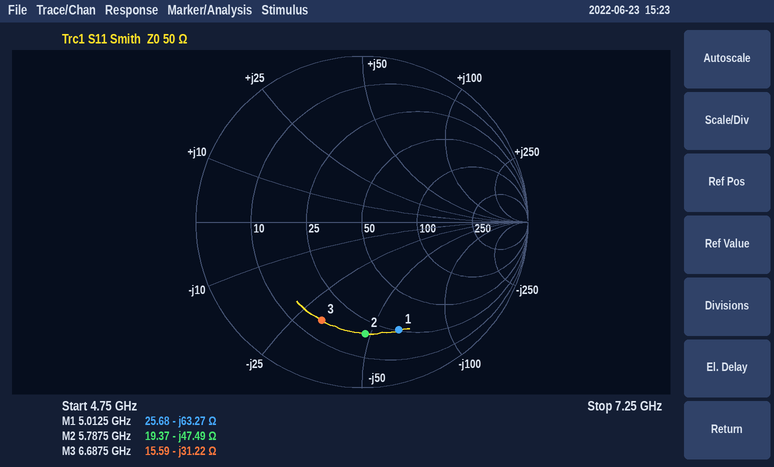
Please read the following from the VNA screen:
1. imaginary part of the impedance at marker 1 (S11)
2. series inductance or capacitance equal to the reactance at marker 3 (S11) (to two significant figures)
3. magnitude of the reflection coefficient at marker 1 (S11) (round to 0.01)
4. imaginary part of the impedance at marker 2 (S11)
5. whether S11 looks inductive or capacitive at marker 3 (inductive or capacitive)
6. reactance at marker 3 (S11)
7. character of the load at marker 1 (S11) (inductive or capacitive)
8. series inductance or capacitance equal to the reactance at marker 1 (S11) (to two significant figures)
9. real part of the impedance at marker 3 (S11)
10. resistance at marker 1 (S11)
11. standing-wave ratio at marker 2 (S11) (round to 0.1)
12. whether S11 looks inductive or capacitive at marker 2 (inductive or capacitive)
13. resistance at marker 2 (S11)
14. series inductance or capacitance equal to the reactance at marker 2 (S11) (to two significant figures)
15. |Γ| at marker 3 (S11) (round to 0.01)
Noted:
-63.27 Ω
760 fF
0.69
-47.49 Ω
capacitive
-31.22 Ω
capacitive
500 fF
15.59 Ω
25.68 Ω
5.1
capacitive
19.37 Ω
580 fF
0.64
